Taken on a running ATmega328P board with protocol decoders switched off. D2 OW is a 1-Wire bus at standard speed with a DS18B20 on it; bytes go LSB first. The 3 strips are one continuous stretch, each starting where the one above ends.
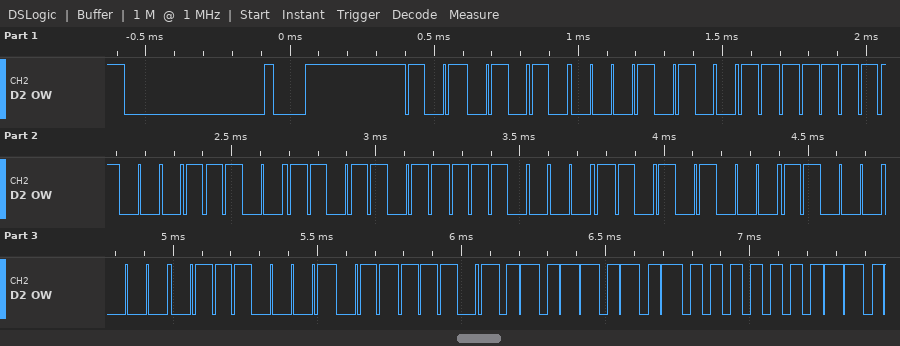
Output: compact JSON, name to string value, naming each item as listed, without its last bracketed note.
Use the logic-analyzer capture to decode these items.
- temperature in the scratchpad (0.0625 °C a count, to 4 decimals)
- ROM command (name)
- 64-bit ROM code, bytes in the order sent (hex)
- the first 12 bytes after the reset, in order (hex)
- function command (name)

{"temperature in the scratchpad": "21.6250 °C", "ROM command": "Match ROM", "64-bit ROM code, bytes in the order sent": "28 FF 38 DB 87 15 03 8E", "the first 12 bytes after the reset, in order": "55 28 FF 38 DB 87 15 03 8E BE 5A 01", "function command": "Read Scratchpad"}
